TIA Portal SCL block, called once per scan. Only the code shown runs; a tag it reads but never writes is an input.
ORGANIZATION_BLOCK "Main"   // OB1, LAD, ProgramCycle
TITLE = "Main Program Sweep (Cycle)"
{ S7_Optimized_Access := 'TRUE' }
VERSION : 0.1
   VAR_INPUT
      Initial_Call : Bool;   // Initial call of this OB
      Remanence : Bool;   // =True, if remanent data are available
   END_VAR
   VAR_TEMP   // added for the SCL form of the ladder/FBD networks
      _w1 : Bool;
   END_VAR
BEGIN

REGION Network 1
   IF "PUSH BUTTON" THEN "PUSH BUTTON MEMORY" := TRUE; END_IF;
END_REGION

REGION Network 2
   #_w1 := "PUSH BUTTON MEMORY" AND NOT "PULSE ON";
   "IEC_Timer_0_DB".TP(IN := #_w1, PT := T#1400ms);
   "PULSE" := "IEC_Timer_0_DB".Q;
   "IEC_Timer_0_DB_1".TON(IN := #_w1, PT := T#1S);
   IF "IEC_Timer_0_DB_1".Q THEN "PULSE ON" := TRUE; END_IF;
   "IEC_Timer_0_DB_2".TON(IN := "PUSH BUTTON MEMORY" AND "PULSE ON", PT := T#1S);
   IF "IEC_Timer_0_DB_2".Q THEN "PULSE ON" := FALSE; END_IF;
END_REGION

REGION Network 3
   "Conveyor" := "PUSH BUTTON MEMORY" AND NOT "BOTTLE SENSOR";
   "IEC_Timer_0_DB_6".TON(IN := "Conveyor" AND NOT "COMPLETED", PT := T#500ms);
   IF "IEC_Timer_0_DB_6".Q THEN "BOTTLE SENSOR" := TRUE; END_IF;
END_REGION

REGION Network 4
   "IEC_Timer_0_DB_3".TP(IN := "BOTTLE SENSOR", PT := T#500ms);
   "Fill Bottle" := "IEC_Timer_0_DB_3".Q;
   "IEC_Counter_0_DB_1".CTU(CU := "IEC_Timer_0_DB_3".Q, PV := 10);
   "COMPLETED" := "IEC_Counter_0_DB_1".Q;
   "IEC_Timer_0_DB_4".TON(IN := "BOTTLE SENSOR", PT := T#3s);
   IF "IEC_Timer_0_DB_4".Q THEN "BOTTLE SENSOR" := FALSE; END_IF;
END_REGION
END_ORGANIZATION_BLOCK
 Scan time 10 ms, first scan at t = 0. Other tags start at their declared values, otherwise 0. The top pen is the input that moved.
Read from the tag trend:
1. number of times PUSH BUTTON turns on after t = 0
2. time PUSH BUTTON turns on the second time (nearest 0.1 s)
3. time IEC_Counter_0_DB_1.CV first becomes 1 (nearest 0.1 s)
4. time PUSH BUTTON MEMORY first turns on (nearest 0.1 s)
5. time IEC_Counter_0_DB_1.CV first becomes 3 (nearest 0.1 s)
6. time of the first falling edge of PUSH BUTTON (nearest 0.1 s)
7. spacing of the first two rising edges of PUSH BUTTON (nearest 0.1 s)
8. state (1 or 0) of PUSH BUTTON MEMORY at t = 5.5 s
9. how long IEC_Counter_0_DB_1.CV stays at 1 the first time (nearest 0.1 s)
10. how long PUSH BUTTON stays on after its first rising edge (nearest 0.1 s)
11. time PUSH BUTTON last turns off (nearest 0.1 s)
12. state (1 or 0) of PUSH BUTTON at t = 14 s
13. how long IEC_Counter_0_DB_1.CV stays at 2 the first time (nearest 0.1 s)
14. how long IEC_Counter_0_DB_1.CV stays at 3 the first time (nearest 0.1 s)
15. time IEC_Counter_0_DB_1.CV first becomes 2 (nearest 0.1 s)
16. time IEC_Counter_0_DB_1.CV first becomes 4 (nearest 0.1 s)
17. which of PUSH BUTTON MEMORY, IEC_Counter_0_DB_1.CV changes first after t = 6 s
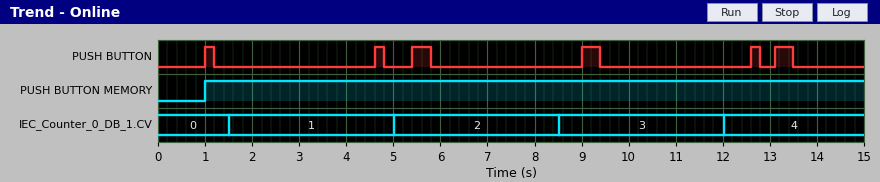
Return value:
6
4.6 s
1.5 s
1.0 s
8.5 s
1.2 s
3.6 s
1
3.5 s
0.2 s
13.5 s
0
3.5 s
3.5 s
5.0 s
12.0 s
IEC_Counter_0_DB_1.CV
